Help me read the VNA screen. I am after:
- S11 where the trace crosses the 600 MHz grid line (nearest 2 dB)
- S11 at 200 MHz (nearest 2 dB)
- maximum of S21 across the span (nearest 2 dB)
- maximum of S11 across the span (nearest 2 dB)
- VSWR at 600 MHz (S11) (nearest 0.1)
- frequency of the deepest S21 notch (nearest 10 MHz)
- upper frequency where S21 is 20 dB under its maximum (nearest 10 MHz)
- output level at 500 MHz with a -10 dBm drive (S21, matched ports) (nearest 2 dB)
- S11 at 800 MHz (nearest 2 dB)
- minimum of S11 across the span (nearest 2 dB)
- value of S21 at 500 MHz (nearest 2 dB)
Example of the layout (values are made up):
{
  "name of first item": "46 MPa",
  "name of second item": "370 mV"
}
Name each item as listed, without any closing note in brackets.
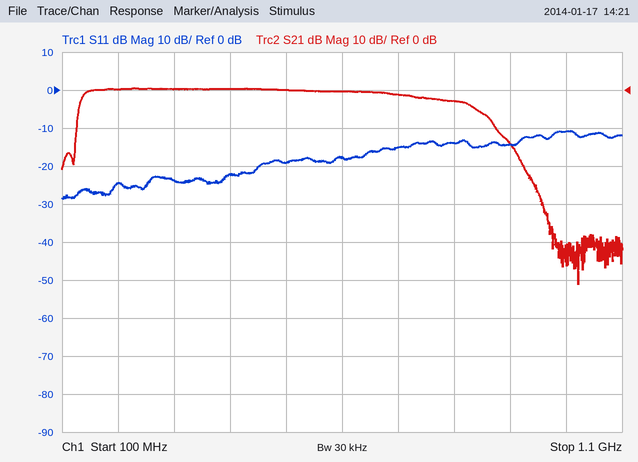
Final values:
{
  "S11 where the trace crosses the 600 MHz grid line": "-18 dB",
  "S11 at 200 MHz": "-24 dB",
  "maximum of S21 across the span": "0 dB",
  "maximum of S11 across the span": "-10 dB",
  "VSWR at 600 MHz (S11)": "1.3",
  "frequency of the deepest S21 notch": "1.02 GHz",
  "upper frequency where S21 is 20 dB under its maximum": "920 MHz",
  "output level at 500 MHz with a -10 dBm drive (S21, matched ports)": "-10 dBm",
  "S11 at 800 MHz": "-14 dB",
  "minimum of S11 across the span": "-28 dB",
  "value of S21 at 500 MHz": "0 dB"
}
